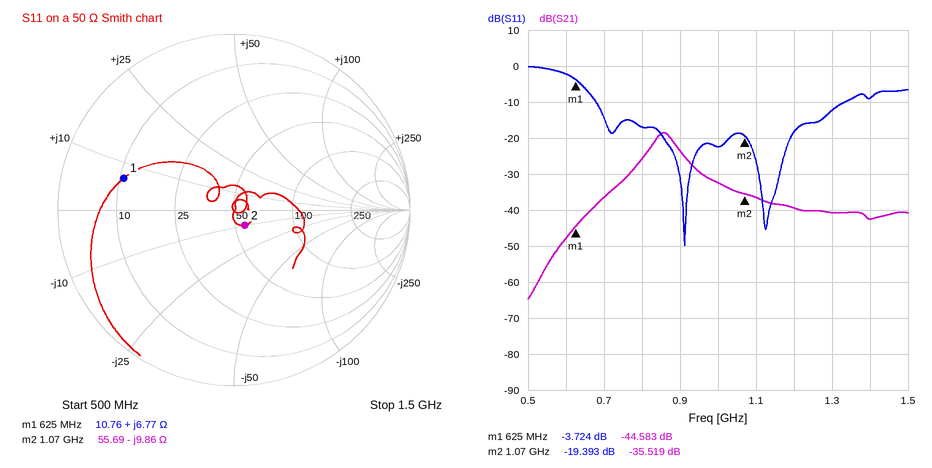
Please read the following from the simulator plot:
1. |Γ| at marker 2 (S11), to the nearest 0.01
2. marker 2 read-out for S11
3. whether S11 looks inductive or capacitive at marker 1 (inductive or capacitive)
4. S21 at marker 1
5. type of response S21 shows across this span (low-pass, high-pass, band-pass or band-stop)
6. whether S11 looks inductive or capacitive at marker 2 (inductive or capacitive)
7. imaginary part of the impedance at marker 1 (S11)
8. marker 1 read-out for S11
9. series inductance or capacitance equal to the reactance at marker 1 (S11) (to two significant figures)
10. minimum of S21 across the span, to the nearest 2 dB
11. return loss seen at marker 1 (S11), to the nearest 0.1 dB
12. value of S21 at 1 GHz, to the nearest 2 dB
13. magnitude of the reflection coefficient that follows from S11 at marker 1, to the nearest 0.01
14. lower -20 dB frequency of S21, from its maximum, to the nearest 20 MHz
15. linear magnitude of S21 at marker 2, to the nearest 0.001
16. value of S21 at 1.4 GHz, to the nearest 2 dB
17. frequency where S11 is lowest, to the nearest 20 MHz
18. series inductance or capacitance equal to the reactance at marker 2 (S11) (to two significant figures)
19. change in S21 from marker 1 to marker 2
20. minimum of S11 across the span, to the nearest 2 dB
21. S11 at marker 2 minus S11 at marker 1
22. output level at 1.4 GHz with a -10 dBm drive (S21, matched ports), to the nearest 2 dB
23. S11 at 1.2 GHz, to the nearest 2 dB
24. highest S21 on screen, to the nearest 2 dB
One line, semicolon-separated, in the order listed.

0.11; -19.393 dB; inductive; -44.583 dB; band-pass; capacitive; +6.77 Ω; -3.724 dB; 1.7 nH; -64 dB; 3.7 dB; -32 dB; 0.65; 680 MHz; 0.017; -42 dB; 920 MHz; 15 pF; 9.064 dB; -50 dB; -15.669 dB; -52 dBm; -18 dB; -18 dB
